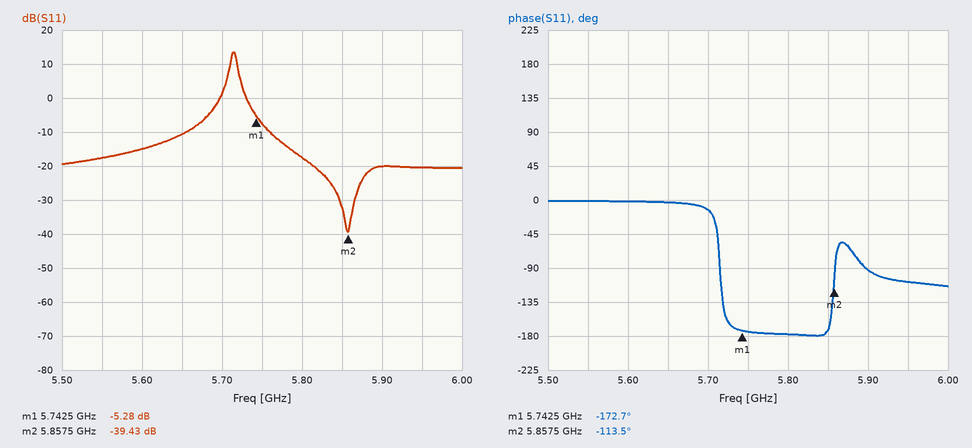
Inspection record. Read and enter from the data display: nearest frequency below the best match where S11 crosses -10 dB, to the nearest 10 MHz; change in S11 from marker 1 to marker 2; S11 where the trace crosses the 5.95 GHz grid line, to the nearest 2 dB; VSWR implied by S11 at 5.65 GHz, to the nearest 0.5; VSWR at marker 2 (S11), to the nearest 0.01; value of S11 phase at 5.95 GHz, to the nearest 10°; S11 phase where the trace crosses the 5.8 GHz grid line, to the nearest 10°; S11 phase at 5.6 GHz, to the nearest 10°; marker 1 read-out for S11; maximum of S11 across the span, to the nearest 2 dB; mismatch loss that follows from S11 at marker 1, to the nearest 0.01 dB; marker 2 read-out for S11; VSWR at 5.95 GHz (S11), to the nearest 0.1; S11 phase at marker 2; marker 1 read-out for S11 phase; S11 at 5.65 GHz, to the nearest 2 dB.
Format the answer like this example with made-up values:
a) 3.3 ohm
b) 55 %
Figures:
a) 5.76 GHz
b) -34.15 dB
c) -20 dB
d) 2.0
e) 1.02
f) -110°
g) -180°
h) 0°
i) -5.28 dB
j) 14 dB
k) 1.53 dB
l) -39.43 dB
m) 1.2
n) -113.5°
o) -172.7°
p) -10 dB
